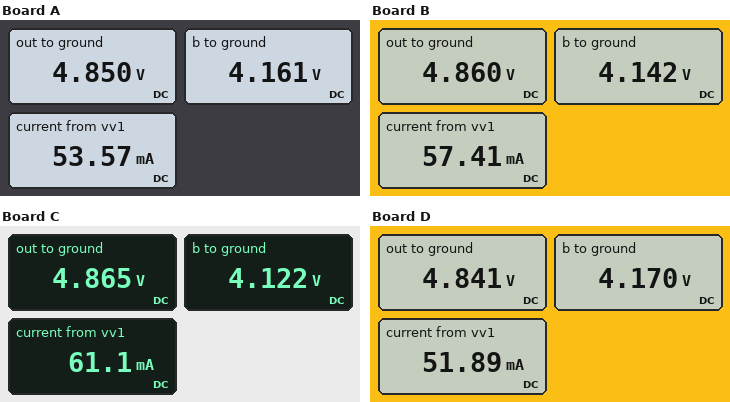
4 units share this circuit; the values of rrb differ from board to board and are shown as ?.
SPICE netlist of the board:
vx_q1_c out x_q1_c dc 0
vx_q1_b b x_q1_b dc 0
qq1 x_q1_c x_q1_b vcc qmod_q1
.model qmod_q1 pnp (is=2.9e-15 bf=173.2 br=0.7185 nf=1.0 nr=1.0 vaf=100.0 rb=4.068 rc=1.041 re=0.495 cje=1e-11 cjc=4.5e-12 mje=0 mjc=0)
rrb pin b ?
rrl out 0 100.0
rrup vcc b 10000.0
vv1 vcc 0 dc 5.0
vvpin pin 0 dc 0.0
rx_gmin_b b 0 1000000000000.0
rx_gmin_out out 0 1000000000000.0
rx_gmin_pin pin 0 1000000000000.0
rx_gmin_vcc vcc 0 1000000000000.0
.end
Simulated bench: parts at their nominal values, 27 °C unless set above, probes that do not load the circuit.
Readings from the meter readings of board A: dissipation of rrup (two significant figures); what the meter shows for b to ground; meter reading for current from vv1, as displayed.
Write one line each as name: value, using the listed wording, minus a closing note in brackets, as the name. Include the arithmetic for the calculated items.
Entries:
dissipation of rrup: (5 V - 4.161 V)^2 / 10 kΩ = 70 µW
what the meter shows for b to ground: 4.161 V
meter reading for current from vv1, as displayed: 53.57 mA
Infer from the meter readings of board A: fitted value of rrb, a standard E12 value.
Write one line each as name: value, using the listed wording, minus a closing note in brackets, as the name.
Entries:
fitted value of rrb, a standard E12 value: 820 Ω
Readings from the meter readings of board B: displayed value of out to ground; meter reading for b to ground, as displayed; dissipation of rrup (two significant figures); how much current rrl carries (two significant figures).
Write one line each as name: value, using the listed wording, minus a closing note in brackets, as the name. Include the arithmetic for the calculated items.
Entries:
displayed value of out to ground: 4.860 V
meter reading for b to ground, as displayed: 4.142 V
dissipation of rrup: (5 V - 4.142 V)^2 / 10 kΩ = 74 µW
how much current rrl carries: (4.86 V) / 100 Ω = 49 mA
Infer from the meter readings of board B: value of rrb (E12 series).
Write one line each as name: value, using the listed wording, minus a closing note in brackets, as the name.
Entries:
value of rrb: 470 Ω
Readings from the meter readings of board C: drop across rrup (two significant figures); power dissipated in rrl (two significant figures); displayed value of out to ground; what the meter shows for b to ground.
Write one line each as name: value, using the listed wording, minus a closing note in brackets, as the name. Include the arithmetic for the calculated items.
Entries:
drop across rrup: 5 V - 4.122 V = 880 mV
power dissipated in rrl: (4.865 V)^2 / 100 Ω = 240 mW
displayed value of out to ground: 4.865 V
what the meter shows for b to ground: 4.122 V
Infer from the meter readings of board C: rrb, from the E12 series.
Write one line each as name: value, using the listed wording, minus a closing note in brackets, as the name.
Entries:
rrb, from the E12 series: 330 Ω
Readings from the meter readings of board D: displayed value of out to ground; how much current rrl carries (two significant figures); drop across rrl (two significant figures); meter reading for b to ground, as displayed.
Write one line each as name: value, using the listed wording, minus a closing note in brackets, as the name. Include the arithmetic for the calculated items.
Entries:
displayed value of out to ground: 4.841 V
how much current rrl carries: (4.841 V) / 100 Ω = 48 mA
drop across rrl: 4.841 V = 4.8 V
meter reading for b to ground, as displayed: 4.170 V
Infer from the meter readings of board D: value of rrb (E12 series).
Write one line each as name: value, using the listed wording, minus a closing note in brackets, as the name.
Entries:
value of rrb: 1.2 kΩ
